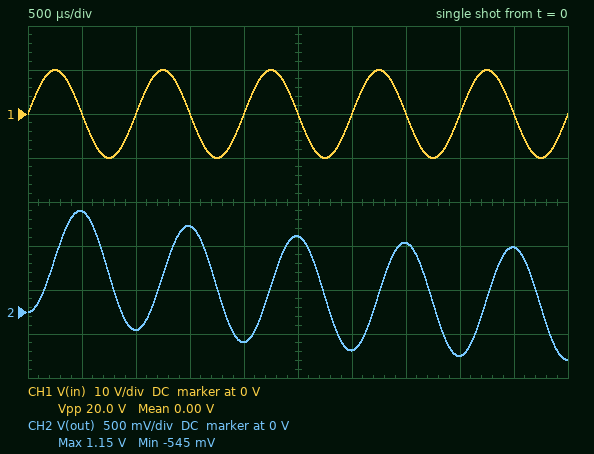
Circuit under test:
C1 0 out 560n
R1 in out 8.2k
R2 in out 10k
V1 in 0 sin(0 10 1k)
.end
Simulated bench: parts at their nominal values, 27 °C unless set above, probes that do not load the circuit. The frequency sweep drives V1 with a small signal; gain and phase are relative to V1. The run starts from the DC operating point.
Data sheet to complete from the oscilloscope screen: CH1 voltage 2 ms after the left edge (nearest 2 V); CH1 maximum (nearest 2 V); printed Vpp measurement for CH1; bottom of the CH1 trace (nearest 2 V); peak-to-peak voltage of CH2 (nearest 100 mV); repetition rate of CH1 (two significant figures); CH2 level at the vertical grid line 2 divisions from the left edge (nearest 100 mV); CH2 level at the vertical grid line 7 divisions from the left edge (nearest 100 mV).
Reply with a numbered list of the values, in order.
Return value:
1. 0 V
2. 10 V
3. 20.0 V
4. -10 V
5. 1.7 V
6. 1.0 kHz
7. -200 mV
8. 800 mV
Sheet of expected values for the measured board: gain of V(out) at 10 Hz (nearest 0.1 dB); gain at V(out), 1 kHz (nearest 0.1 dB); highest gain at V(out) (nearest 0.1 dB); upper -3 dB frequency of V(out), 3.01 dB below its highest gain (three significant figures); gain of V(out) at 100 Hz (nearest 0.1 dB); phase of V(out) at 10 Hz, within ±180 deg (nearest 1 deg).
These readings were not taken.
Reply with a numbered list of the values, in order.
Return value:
1. -0.1 dB
2. -24.0 dB
3. 0 dB
4. 63.1 Hz
5. -5.5 dB
6. -9 deg
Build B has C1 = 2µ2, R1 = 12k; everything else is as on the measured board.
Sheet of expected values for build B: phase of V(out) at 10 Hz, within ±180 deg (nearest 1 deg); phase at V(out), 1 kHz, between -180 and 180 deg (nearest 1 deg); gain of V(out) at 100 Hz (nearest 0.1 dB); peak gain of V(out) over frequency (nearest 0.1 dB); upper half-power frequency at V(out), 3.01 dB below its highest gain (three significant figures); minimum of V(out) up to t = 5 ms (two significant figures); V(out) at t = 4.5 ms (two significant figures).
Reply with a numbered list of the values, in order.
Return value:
1. -37 deg
2. -89 deg
3. -17.6 dB
4. 0 dB
5. 13.3 Hz
6. -45 mV
7. 220 mV
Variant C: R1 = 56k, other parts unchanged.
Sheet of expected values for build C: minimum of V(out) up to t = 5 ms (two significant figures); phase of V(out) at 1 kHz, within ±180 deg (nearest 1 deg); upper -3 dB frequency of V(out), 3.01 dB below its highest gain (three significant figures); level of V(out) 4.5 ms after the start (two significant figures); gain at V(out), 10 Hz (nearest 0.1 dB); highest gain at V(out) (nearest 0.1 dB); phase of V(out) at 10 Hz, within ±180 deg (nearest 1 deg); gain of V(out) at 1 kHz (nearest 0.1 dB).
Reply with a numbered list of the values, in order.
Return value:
1. -220 mV
2. -88 deg
3. 33.5 Hz
4. 460 mV
5. -0.4 dB
6. 0 dB
7. -17 deg
8. -29.5 dB
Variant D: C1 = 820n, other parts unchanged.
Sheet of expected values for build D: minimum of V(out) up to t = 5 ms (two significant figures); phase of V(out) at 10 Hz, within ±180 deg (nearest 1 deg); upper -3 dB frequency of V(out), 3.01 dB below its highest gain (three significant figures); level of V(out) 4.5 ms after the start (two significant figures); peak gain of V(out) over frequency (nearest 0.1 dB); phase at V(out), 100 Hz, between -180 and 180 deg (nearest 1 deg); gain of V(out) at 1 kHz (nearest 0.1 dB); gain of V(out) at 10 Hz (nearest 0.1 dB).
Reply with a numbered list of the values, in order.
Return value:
1. -320 mV
2. -13 deg
3. 43.1 Hz
4. 560 mV
5. 0 dB
6. -67 deg
7. -27.3 dB
8. -0.2 dB
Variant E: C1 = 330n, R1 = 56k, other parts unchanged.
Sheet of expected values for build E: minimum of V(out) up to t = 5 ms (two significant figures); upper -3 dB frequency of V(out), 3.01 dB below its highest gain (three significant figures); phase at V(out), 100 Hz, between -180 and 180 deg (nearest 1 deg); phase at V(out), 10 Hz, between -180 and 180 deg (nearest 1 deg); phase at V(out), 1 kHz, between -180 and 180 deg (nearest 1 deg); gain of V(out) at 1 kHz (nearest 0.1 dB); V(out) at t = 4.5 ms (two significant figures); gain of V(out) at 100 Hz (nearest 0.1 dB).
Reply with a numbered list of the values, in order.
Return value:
1. -470 mV
2. 56.8 Hz
3. -60 deg
4. -10 deg
5. -87 deg
6. -24.9 dB
7. 680 mV
8. -6.1 dB
